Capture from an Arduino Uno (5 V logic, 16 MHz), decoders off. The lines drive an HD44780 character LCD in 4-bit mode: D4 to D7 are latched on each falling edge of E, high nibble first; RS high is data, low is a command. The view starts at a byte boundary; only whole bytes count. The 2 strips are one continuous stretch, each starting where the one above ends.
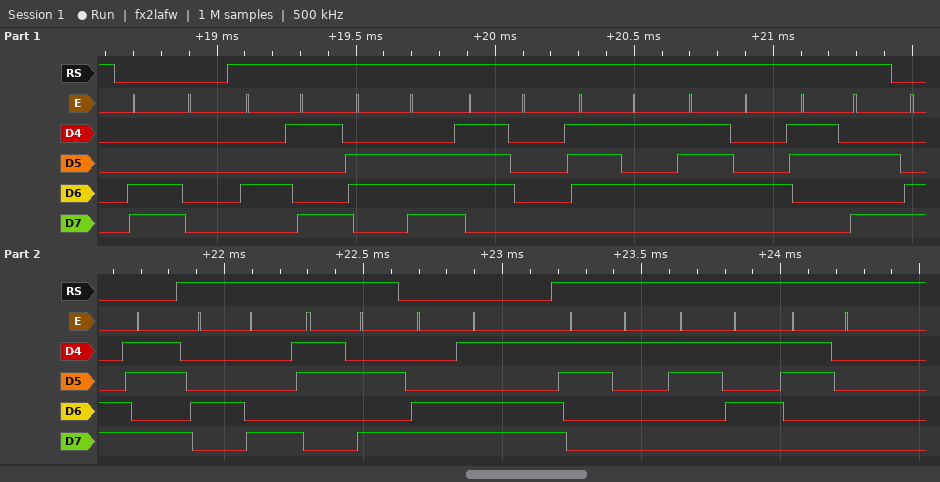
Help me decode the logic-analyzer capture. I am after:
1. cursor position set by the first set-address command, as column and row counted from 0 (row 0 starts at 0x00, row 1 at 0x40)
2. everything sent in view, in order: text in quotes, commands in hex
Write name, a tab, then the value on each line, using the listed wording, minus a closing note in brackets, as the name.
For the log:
cursor position set by the first set-address command, as column and row counted from 0	column 0, row 1
everything sent in view, in order: text in quotes, commands in hex	0xC0 "Input:" 0xCB "H:" 0xCD "150"
